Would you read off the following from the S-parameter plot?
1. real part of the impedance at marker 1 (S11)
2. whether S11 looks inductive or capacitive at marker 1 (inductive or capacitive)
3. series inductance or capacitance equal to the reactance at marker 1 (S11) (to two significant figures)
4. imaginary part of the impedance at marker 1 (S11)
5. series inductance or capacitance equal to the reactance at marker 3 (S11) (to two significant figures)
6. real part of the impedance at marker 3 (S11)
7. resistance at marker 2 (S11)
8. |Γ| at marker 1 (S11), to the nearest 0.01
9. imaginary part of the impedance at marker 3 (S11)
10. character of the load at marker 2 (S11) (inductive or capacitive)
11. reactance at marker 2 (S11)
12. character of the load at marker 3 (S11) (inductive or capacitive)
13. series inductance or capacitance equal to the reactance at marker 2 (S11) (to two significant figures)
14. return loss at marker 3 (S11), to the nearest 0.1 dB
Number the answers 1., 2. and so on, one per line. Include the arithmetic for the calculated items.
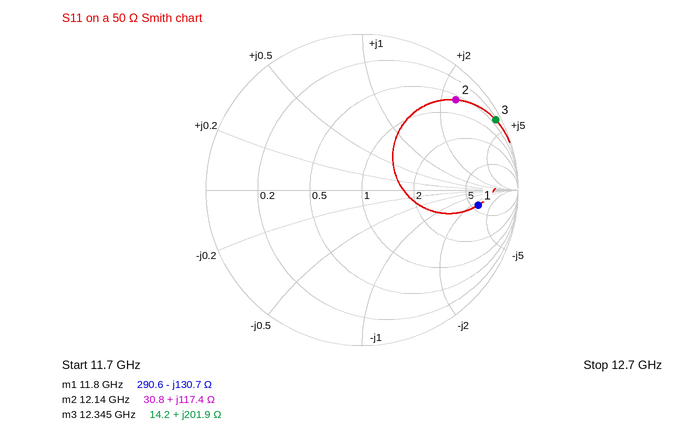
1. 290.6 Ω
2. capacitive
3. C = 1/(2π × 11.8 GHz × 130.7 Ω) ≈ 103 fF, so 100 fF to two significant figures
4. -130.7 Ω
5. L = 201.9 Ω/(2π × 12.345 GHz) ≈ 2.6 nH
6. 14.2 Ω
7. 30.8 Ω
8. 0.75
9. +201.9 Ω
10. inductive
11. +117.4 Ω
12. inductive
13. L = 117.4 Ω/(2π × 12.14 GHz) ≈ 1.5 nH
14. 0.3 dB
